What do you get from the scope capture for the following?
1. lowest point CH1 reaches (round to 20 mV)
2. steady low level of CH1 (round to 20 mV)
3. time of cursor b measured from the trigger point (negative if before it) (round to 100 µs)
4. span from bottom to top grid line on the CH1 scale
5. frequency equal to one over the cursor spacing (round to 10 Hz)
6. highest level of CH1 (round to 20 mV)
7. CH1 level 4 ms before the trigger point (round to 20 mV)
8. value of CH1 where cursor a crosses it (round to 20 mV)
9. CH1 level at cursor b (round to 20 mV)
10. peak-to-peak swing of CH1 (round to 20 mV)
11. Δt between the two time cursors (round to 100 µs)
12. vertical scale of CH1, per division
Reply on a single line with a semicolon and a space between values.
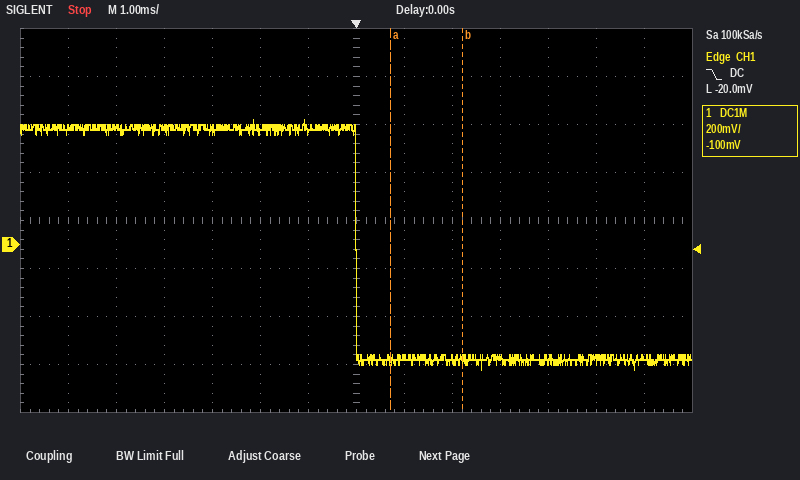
-520 mV; -480 mV; +2.2 ms; 1.6 V; 670 Hz; 520 mV; 480 mV; -480 mV; -480 mV; 1.04 V; 1.5 ms; 200 mV
